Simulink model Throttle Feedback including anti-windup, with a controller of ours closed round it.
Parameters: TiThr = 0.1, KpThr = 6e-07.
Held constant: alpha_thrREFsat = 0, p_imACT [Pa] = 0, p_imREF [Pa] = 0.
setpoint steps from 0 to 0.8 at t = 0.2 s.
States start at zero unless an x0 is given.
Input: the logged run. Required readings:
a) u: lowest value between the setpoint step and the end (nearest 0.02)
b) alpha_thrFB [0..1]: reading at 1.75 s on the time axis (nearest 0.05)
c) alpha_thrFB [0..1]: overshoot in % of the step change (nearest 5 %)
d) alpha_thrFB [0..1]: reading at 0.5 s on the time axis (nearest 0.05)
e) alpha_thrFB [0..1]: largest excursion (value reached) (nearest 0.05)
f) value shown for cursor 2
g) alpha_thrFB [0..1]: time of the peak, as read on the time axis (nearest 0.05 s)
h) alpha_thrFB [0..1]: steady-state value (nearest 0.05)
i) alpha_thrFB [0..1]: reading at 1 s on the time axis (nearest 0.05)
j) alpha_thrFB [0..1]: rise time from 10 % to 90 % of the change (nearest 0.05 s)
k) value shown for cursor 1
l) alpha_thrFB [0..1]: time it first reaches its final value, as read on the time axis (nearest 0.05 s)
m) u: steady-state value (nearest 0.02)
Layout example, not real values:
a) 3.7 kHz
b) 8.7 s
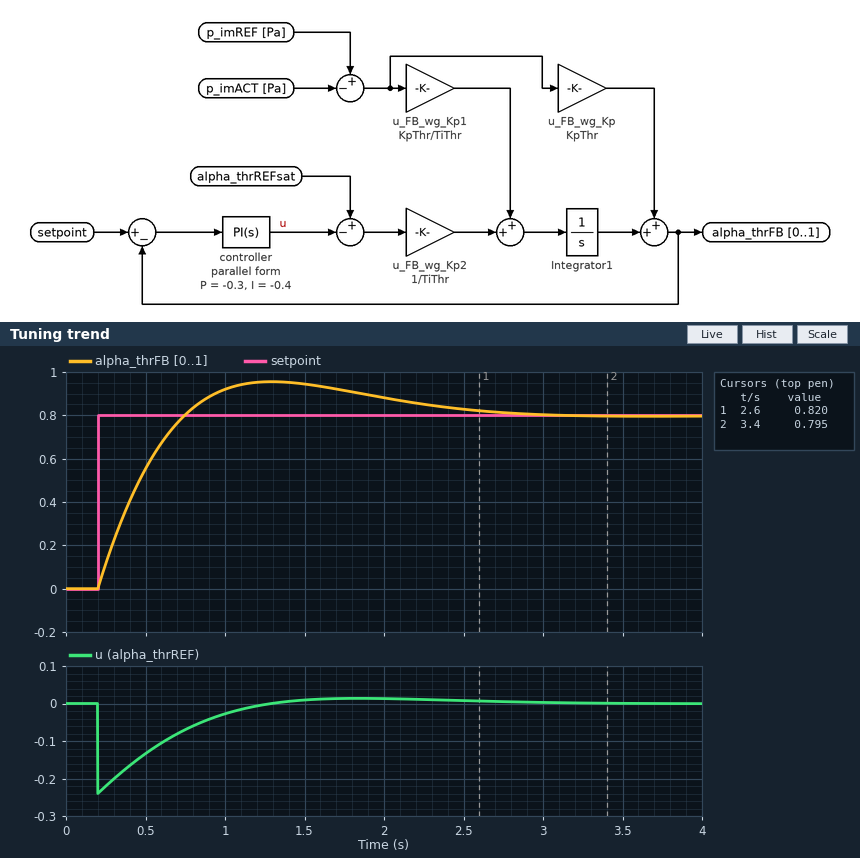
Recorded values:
a) -0.24
b) 0.90
c) 20 %
d) 0.55
e) 0.95
f) 0.795
g) 1.30 s
h) 0.80
i) 0.90
j) 0.40 s
k) 0.820
l) 0.75 s
m) 0.00
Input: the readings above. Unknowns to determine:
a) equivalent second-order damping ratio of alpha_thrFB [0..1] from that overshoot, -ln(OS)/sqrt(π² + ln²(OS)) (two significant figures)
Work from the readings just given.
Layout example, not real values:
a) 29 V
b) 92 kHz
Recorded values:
a) 0.46
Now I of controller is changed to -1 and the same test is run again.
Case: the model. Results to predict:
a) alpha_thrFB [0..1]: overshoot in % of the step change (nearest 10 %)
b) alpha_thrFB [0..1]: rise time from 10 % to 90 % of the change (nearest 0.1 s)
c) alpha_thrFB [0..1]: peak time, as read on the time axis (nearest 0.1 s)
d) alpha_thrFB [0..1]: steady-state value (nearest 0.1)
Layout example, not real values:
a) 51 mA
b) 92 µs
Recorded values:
a) 30 %
b) 0.3 s
c) 1.0 s
d) 0.8
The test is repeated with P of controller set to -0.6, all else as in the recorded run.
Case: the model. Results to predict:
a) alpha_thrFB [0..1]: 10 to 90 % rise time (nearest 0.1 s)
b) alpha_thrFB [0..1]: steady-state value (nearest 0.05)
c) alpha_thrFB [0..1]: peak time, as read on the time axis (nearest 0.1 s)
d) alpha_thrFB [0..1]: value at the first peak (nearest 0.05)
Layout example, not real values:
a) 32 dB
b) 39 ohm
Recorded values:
a) 0.3 s
b) 0.80
c) 1.1 s
d) 0.85
